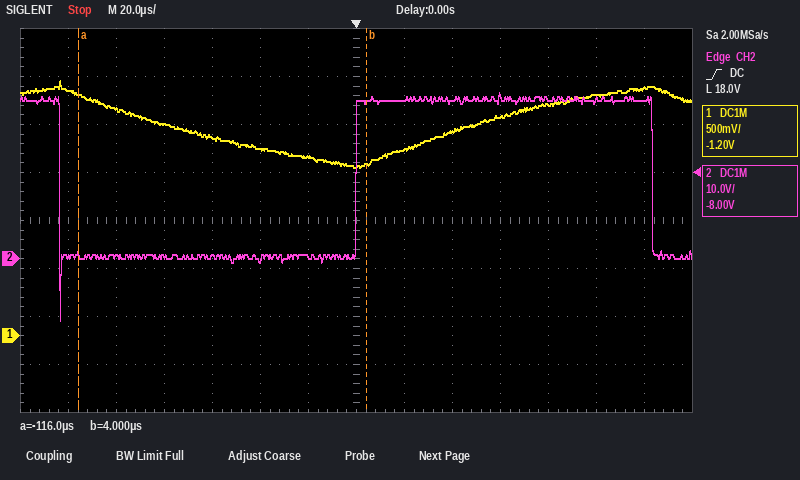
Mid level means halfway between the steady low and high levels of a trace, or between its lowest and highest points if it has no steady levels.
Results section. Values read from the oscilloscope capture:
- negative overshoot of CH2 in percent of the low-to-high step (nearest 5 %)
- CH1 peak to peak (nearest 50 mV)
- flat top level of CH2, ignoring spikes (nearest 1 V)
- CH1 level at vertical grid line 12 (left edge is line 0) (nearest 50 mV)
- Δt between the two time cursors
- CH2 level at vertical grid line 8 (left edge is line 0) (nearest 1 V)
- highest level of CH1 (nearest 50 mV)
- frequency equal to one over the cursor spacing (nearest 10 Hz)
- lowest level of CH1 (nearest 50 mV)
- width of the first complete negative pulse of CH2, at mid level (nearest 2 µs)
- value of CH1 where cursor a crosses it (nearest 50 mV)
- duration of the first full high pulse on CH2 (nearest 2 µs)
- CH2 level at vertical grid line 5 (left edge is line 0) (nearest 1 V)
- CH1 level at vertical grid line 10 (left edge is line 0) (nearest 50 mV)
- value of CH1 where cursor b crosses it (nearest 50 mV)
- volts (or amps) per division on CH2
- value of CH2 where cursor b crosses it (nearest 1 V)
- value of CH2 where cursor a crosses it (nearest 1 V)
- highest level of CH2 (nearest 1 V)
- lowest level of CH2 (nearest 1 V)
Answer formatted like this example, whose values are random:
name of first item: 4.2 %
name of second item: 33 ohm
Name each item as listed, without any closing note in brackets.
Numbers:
negative overshoot of CH2 in percent of the low-to-high step: 40 %
CH1 peak to peak: 900 mV
flat top level of CH2, ignoring spikes: 33 V
CH1 level at vertical grid line 12 (left edge is line 0): 2.50 V
Δt between the two time cursors: 120 µs
CH2 level at vertical grid line 8 (left edge is line 0): 33 V
highest level of CH1: 2.65 V
frequency equal to one over the cursor spacing: 8.33 kHz
lowest level of CH1: 1.75 V
width of the first complete negative pulse of CH2, at mid level: 124 µs
value of CH1 where cursor a crosses it: 2.50 V
duration of the first full high pulse on CH2: 124 µs
CH2 level at vertical grid line 5 (left edge is line 0): 0 V
CH1 level at vertical grid line 10 (left edge is line 0): 2.30 V
value of CH1 where cursor b crosses it: 1.80 V
volts (or amps) per division on CH2: 10 V
value of CH2 where cursor b crosses it: 33 V
value of CH2 where cursor a crosses it: 1 V
highest level of CH2: 35 V
lowest level of CH2: -13 V
